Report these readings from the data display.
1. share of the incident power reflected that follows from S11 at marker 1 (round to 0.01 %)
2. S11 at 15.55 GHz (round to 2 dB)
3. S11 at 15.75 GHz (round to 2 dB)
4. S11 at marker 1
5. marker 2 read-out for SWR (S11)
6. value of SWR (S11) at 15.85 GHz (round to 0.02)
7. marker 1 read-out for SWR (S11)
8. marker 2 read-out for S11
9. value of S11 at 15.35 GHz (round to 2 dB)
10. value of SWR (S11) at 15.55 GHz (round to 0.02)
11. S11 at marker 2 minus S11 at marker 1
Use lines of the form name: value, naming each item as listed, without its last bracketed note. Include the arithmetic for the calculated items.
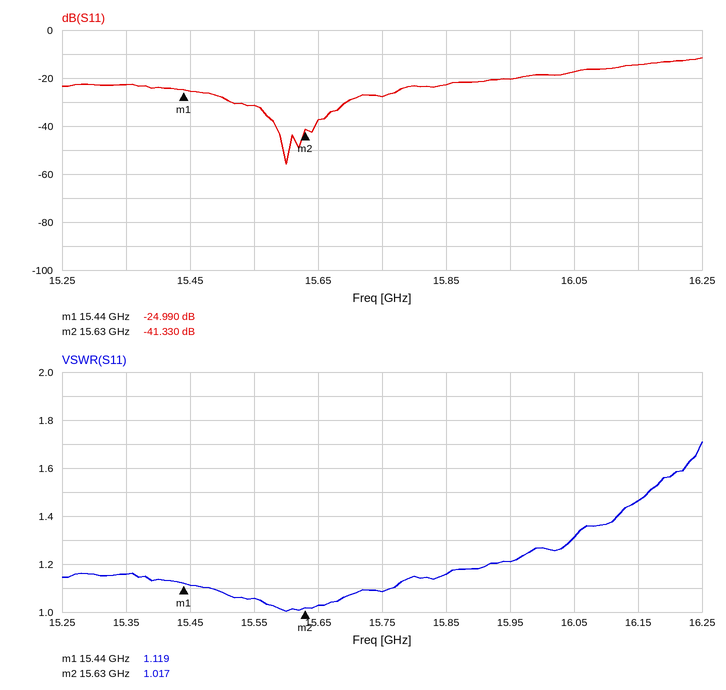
share of the incident power reflected that follows from S11 at marker 1: 10^(-24.99/10) ≈ 0.32 %
S11 at 15.55 GHz: -32 dB
S11 at 15.75 GHz: -28 dB
S11 at marker 1: -24.990 dB
marker 2 read-out for SWR: 1.017
value of SWR (S11) at 15.85 GHz: 1.16
marker 1 read-out for SWR: 1.119
marker 2 read-out for S11: -41.330 dB
value of S11 at 15.35 GHz: -22 dB
value of SWR (S11) at 15.55 GHz: 1.06
S11 at marker 2 minus S11 at marker 1: -41.33 − (-24.99) = -16.340 dB
